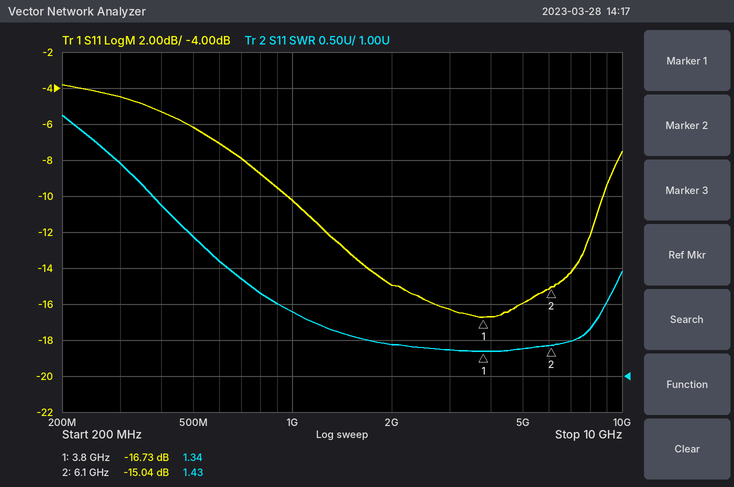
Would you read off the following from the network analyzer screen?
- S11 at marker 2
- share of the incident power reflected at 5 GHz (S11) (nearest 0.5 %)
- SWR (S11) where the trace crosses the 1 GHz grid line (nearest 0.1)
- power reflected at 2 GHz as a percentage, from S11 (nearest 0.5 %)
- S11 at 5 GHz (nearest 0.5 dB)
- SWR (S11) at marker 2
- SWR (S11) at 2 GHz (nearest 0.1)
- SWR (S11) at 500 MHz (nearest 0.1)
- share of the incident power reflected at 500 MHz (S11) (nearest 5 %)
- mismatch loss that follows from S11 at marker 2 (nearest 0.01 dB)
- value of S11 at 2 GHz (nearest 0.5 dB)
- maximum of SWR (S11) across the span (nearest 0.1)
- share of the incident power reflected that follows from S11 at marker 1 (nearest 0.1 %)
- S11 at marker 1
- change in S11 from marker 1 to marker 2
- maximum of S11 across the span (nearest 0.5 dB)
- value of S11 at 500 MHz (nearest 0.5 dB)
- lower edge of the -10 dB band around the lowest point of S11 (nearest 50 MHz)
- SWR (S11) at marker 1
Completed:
-15.04 dB
2.5 %
1.9
3.0 %
-16.0 dB
1.43
1.4
2.9
25 %
0.14 dB
-15.0 dB
4.6
2.1 %
-16.73 dB
1.69 dB
-4.0 dB
-6.0 dB
950 MHz
1.34
